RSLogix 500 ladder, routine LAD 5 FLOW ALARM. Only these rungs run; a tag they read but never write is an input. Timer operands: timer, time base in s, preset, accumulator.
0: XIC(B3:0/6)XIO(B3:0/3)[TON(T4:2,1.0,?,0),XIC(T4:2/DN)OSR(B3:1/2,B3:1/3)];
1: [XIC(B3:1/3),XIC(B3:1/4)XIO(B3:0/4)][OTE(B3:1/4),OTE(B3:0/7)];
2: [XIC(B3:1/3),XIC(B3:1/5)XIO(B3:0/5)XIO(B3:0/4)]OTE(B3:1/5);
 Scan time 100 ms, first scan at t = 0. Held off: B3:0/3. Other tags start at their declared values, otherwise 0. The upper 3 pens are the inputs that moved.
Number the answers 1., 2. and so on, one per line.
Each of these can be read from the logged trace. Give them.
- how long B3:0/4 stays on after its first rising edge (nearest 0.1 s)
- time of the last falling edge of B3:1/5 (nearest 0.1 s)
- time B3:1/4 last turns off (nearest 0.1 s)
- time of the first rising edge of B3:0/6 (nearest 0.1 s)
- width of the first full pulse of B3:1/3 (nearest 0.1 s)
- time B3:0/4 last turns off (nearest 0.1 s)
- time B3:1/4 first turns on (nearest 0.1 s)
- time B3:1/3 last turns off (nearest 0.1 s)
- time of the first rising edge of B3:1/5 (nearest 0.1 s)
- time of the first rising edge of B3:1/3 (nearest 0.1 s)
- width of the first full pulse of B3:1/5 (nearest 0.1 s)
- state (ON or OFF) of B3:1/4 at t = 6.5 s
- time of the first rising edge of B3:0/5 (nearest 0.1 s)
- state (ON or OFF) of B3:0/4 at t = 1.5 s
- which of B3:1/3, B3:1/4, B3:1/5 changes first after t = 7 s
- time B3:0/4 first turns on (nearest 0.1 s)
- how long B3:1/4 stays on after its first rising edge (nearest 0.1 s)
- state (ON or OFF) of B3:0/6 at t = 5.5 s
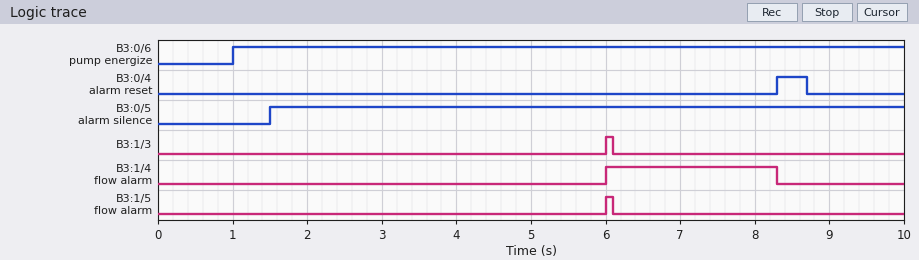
1. 0.4 s
2. 6.1 s
3. 8.3 s
4. 1.0 s
5. 0.1 s
6. 8.7 s
7. 6.0 s
8. 6.1 s
9. 6.0 s
10. 6.0 s
11. 0.1 s
12. ON
13. 1.5 s
14. OFF
15. B3:1/4
16. 8.3 s
17. 2.3 s
18. ON
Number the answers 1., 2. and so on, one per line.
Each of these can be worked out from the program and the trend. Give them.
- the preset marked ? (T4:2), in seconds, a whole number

1. 5 s
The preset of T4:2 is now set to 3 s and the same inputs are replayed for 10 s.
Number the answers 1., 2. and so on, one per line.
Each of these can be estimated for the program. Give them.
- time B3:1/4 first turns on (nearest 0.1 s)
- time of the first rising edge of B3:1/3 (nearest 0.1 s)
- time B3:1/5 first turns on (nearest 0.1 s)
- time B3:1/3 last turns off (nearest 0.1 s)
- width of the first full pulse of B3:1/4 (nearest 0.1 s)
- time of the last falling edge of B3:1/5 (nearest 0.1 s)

1. 4.0 s
2. 4.0 s
3. 4.0 s
4. 4.1 s
5. 4.3 s
6. 4.1 s
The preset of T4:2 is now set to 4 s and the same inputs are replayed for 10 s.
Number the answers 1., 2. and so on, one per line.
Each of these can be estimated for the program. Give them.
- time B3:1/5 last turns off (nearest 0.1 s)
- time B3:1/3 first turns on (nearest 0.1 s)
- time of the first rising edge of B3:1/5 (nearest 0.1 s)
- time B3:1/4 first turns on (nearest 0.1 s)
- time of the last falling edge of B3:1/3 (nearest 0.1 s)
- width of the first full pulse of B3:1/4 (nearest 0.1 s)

1. 5.1 s
2. 5.0 s
3. 5.0 s
4. 5.0 s
5. 5.1 s
6. 3.3 s
